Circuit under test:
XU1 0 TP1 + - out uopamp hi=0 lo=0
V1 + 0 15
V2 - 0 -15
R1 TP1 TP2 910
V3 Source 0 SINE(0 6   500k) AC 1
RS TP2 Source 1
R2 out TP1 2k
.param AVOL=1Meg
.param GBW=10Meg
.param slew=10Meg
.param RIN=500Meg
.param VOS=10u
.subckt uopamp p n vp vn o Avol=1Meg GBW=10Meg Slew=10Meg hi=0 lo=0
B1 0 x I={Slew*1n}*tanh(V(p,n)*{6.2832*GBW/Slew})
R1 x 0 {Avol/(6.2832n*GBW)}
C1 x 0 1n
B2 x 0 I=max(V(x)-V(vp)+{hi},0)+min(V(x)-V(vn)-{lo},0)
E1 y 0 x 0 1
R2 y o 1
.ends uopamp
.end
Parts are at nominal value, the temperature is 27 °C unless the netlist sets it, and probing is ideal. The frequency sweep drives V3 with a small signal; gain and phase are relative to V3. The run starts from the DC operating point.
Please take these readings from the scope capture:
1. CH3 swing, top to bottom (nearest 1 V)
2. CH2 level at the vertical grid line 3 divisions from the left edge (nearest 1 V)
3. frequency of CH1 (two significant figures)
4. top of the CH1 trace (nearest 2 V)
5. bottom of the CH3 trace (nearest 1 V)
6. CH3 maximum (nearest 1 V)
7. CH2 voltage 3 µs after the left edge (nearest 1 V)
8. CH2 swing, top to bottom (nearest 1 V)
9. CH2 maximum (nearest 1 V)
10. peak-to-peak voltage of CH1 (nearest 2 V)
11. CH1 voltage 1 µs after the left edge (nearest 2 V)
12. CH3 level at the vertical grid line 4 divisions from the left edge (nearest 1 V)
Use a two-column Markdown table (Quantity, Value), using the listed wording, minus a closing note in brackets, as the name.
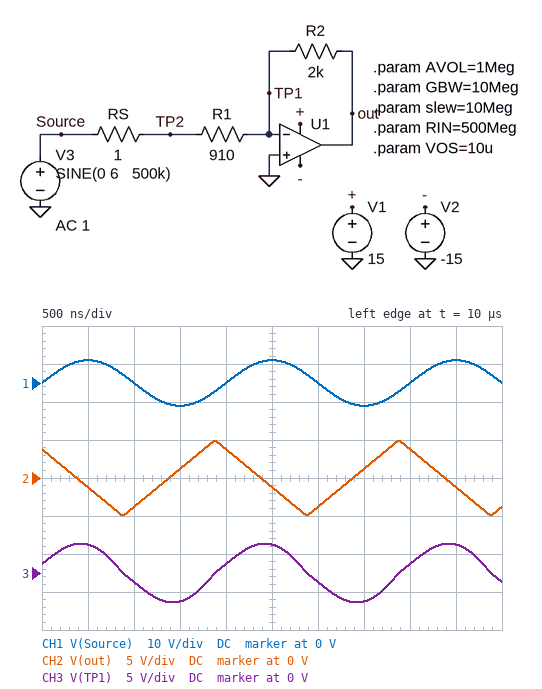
| Quantity | Value |
|---|---|
| CH3 swing, top to bottom | 8 V |
| CH2 level at the vertical grid line 3 divisions from the left edge | 1 V |
| frequency of CH1 | 500 kHz |
| top of the CH1 trace | 6 V |
| bottom of the CH3 trace | -4 V |
| CH3 maximum | 4 V |
| CH2 voltage 3 µs after the left edge | -4 V |
| CH2 swing, top to bottom | 10 V |
| CH2 maximum | 5 V |
| peak-to-peak voltage of CH1 | 12 V |
| CH1 voltage 1 µs after the left edge | 0 V |
| CH3 level at the vertical grid line 4 divisions from the left edge | 1 V |
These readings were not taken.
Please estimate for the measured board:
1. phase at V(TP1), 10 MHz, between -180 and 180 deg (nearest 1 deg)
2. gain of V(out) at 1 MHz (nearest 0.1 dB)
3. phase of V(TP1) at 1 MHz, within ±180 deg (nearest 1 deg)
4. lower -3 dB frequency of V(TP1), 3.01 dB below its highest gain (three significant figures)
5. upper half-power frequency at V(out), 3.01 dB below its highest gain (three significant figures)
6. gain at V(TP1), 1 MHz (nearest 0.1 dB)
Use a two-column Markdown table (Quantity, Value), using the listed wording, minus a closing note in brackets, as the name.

| Quantity | Value |
|---|---|
| phase at V(TP1), 10 MHz, between -180 and 180 deg | 17 deg |
| gain of V(out) at 1 MHz | 6.4 dB |
| phase of V(TP1) at 1 MHz, within ±180 deg | 72 deg |
| lower -3 dB frequency of V(TP1), 3.01 dB below its highest gain | 3.13 MHz |
| upper half-power frequency at V(out), 3.01 dB below its highest gain | 3.13 MHz |
| gain at V(TP1), 1 MHz | -13.6 dB |
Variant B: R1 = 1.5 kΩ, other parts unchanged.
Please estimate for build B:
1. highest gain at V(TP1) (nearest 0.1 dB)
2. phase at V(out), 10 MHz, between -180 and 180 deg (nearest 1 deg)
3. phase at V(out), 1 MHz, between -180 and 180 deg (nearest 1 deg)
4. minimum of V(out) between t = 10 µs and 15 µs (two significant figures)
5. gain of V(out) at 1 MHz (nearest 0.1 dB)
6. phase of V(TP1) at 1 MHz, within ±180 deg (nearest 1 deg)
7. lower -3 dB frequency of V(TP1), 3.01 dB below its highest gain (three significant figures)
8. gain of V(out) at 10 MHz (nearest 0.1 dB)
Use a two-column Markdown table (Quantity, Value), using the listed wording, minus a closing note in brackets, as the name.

| Quantity | Value |
|---|---|
| highest gain at V(TP1) | -4.9 dB |
| phase at V(out), 10 MHz, between -180 and 180 deg | 113 deg |
| phase at V(out), 1 MHz, between -180 and 180 deg | 167 deg |
| minimum of V(out) between t = 10 µs and 15 µs | -4.9 V |
| gain of V(out) at 1 MHz | 2.3 dB |
| phase of V(TP1) at 1 MHz, within ±180 deg | 77 deg |
| lower -3 dB frequency of V(TP1), 3.01 dB below its highest gain | 4.29 MHz |
| gain of V(out) at 10 MHz | -5.6 dB |
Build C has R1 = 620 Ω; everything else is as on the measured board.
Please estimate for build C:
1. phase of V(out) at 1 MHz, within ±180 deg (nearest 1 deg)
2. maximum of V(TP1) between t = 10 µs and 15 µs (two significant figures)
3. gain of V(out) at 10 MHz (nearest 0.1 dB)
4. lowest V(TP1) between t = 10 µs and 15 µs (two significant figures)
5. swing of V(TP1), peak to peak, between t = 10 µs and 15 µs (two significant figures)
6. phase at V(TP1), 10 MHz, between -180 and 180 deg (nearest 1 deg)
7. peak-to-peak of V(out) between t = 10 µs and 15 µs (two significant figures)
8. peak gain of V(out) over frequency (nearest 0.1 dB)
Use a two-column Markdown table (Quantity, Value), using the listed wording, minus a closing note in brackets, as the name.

| Quantity | Value |
|---|---|
| phase of V(out) at 1 MHz, within ±180 deg | 157 deg |
| maximum of V(TP1) between t = 10 µs and 15 µs | 4.4 V |
| gain of V(out) at 10 MHz | -2.6 dB |
| lowest V(TP1) between t = 10 µs and 15 µs | -4.5 V |
| swing of V(TP1), peak to peak, between t = 10 µs and 15 µs | 8.9 V |
| phase at V(TP1), 10 MHz, between -180 and 180 deg | 13 deg |
| peak-to-peak of V(out) between t = 10 µs and 15 µs | 9.9 V |
| peak gain of V(out) over frequency | 10.2 dB |
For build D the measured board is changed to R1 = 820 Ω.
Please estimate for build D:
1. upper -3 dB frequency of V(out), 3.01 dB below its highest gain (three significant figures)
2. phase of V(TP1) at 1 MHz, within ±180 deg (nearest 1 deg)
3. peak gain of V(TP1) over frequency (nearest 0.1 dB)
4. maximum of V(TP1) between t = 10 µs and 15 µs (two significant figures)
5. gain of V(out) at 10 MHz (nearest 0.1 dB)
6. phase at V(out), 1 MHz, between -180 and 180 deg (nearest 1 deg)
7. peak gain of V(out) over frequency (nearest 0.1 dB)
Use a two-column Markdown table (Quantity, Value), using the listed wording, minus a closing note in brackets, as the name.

| Quantity | Value |
|---|---|
| upper -3 dB frequency of V(out), 3.01 dB below its highest gain | 2.91 MHz |
| phase of V(TP1) at 1 MHz, within ±180 deg | 71 deg |
| peak gain of V(TP1) over frequency | -3.0 dB |
| maximum of V(TP1) between t = 10 µs and 15 µs | 4.0 V |
| gain of V(out) at 10 MHz | -3.3 dB |
| phase at V(out), 1 MHz, between -180 and 180 deg | 161 deg |
| peak gain of V(out) over frequency | 7.7 dB |
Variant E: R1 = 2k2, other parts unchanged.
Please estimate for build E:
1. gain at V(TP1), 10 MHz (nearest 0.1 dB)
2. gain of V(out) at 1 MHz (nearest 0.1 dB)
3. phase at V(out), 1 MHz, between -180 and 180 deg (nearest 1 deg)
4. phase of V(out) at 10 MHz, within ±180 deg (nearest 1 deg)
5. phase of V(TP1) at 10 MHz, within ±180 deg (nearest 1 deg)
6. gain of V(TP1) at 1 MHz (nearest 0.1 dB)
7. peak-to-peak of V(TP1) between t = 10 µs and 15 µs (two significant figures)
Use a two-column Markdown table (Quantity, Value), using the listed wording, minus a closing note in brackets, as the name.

| Quantity | Value |
|---|---|
| gain at V(TP1), 10 MHz | -7.5 dB |
| gain of V(out) at 1 MHz | -1.0 dB |
| phase at V(out), 1 MHz, between -180 and 180 deg | 169 deg |
| phase of V(out) at 10 MHz, within ±180 deg | 118 deg |
| phase of V(TP1) at 10 MHz, within ±180 deg | 28 deg |
| gain of V(TP1) at 1 MHz | -21.0 dB |
| peak-to-peak of V(TP1) between t = 10 µs and 15 µs | 3.4 V |
